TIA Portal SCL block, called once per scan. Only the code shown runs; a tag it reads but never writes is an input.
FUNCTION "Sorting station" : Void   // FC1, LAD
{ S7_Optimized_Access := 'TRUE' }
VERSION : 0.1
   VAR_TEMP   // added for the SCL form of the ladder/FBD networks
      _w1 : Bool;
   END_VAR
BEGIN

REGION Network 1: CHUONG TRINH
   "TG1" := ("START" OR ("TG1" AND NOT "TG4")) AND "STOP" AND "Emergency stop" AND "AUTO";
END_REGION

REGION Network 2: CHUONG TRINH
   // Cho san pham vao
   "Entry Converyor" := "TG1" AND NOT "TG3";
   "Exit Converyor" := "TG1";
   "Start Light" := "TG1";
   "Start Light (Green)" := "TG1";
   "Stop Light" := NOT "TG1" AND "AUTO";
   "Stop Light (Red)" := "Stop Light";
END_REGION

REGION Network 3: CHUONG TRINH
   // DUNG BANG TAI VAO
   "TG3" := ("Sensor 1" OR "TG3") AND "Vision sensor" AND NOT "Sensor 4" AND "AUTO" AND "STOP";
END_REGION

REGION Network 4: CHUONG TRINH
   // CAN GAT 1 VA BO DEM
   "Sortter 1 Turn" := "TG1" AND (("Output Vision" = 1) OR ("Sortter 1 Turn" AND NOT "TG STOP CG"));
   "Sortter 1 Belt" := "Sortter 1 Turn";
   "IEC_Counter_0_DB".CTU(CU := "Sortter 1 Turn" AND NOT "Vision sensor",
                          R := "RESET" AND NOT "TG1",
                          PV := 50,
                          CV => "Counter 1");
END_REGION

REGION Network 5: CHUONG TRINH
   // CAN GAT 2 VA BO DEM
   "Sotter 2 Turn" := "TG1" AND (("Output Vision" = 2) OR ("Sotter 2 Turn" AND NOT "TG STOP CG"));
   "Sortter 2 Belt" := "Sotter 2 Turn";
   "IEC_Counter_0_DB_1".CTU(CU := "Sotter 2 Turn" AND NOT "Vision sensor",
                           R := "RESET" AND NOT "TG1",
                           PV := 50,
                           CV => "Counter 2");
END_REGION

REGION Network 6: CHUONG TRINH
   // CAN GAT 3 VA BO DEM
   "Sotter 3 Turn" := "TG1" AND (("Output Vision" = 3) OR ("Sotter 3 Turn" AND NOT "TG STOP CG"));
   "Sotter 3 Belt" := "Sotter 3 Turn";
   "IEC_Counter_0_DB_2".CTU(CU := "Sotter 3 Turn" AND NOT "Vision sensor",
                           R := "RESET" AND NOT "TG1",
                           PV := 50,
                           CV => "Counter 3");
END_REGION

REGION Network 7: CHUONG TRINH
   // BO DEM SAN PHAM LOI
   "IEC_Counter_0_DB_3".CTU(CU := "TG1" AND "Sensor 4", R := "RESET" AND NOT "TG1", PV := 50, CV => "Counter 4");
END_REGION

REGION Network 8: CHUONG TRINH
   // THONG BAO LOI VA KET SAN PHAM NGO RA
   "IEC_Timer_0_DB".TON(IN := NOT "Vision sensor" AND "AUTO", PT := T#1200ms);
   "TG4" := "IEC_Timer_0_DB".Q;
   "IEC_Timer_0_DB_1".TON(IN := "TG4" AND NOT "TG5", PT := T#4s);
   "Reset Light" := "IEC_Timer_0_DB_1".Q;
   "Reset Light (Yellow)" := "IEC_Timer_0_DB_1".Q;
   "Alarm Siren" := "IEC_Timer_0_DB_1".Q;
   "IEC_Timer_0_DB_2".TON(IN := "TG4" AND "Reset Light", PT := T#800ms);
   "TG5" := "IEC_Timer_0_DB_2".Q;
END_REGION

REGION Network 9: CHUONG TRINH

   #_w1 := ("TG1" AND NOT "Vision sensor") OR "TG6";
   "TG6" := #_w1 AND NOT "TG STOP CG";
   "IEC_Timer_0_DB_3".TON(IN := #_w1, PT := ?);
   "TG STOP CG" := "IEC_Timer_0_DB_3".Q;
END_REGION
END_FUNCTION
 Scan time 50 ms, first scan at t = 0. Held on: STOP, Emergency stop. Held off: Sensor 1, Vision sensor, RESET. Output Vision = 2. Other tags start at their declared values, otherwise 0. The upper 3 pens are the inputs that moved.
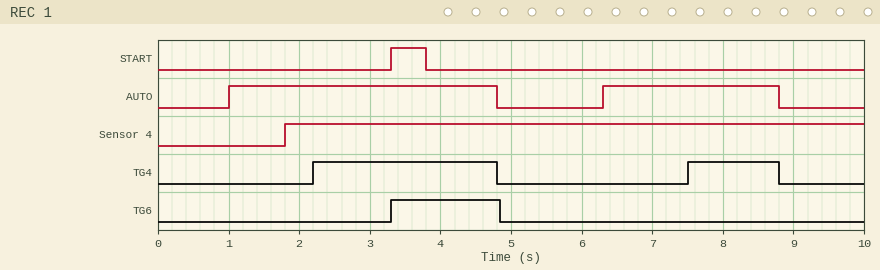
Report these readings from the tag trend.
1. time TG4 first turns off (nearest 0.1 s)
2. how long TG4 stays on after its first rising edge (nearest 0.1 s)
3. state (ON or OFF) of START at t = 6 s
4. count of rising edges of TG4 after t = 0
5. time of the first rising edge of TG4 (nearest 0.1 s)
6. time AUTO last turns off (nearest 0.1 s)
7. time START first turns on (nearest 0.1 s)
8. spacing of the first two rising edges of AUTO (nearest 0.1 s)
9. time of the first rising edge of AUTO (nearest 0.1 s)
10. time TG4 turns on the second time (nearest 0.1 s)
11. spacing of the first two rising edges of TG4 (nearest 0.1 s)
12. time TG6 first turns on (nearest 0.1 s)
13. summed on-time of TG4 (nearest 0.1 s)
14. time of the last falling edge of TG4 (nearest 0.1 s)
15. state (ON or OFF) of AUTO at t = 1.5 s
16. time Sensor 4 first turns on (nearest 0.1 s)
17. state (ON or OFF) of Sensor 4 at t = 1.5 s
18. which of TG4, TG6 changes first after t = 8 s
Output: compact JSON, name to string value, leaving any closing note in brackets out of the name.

{"time TG4 first turns off": "4.8 s", "how long TG4 stays on after its first rising edge": "2.6 s", "state (ON or OFF) of START at t = 6 s": "OFF", "count of rising edges of TG4 after t = 0": "2", "time of the first rising edge of TG4": "2.2 s", "time AUTO last turns off": "8.8 s", "time START first turns on": "3.3 s", "spacing of the first two rising edges of AUTO": "5.3 s", "time of the first rising edge of AUTO": "1.0 s", "time TG4 turns on the second time": "7.5 s", "spacing of the first two rising edges of TG4": "5.3 s", "time TG6 first turns on": "3.3 s", "summed on-time of TG4": "3.9 s", "time of the last falling edge of TG4": "8.8 s", "state (ON or OFF) of AUTO at t = 1.5 s": "ON", "time Sensor 4 first turns on": "1.8 s", "state (ON or OFF) of Sensor 4 at t = 1.5 s": "OFF", "which of TG4, TG6 changes first after t = 8 s": "TG4"}
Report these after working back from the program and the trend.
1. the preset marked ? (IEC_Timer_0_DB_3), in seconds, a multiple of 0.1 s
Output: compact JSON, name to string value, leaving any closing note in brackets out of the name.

{"the preset marked ? (IEC_Timer_0_DB_3), in seconds, a multiple of 0.1 s": "1.5 s"}
